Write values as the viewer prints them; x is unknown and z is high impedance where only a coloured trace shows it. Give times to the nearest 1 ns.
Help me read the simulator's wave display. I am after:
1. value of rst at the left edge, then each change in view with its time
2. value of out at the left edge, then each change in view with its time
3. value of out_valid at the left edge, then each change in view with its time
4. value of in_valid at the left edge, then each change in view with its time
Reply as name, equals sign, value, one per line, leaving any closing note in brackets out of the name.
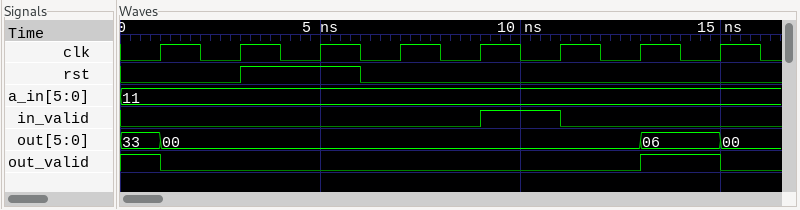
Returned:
value of rst at the left edge, then each change in view with its time = 0, 1 at 3 ns, 0 at 6 ns
value of out at the left edge, then each change in view with its time = 33, 00 at 1 ns, 06 at 13 ns, 00 at 15 ns
value of out_valid at the left edge, then each change in view with its time = 1, 0 at 1 ns, 1 at 13 ns, 0 at 15 ns
value of in_valid at the left edge, then each change in view with its time = 0, 1 at 9 ns, 0 at 11 ns
